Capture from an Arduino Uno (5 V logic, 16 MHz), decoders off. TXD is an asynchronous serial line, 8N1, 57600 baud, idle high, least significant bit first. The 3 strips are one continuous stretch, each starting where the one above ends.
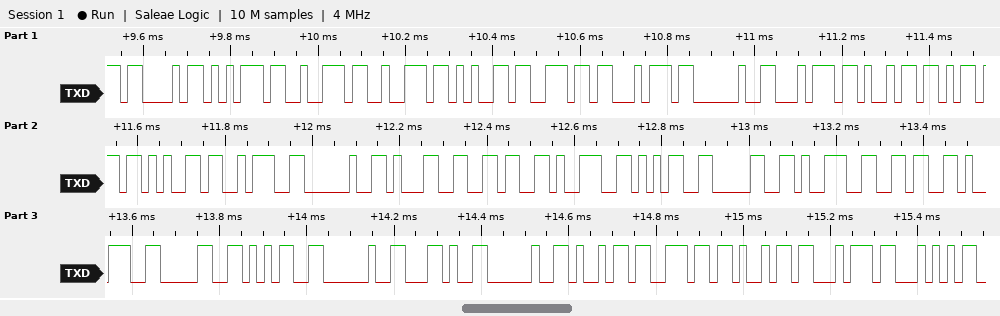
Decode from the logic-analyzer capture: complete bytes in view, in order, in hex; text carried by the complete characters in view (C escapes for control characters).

43 75 72 72 65 6E 74 20 74 69 6D 65 3A 20 31 36 39 35 30 39 36 39 30 35 20 2C 20 69 6E 69 74 54
"Current time: 1695096905 , initT"
